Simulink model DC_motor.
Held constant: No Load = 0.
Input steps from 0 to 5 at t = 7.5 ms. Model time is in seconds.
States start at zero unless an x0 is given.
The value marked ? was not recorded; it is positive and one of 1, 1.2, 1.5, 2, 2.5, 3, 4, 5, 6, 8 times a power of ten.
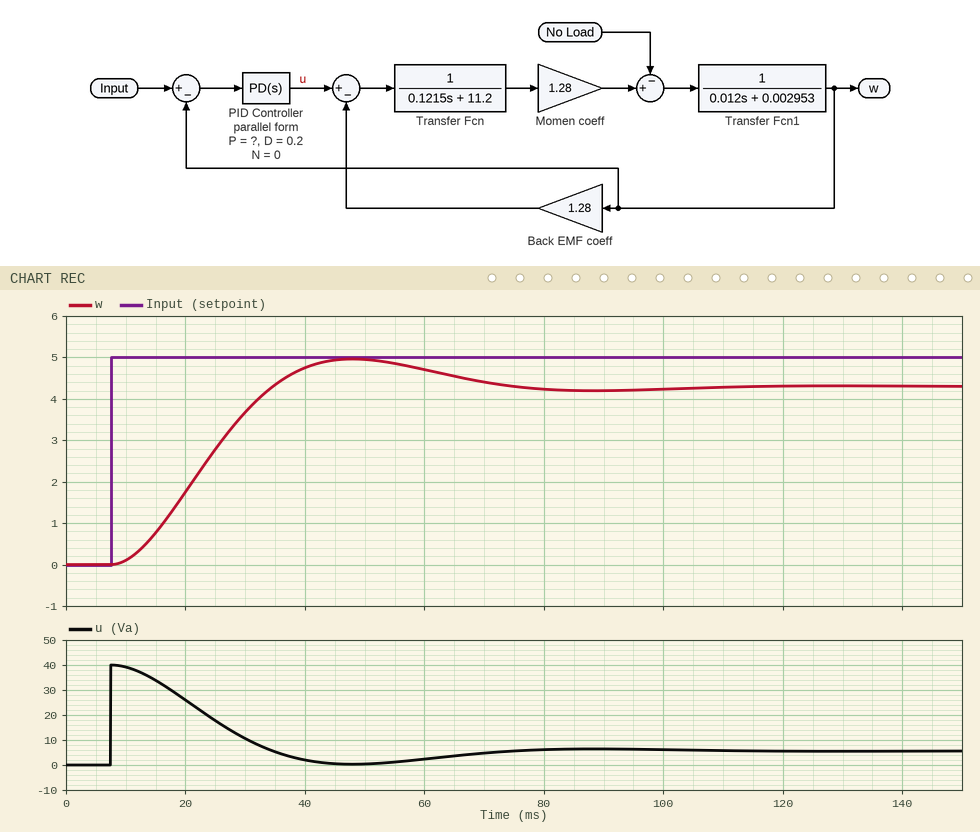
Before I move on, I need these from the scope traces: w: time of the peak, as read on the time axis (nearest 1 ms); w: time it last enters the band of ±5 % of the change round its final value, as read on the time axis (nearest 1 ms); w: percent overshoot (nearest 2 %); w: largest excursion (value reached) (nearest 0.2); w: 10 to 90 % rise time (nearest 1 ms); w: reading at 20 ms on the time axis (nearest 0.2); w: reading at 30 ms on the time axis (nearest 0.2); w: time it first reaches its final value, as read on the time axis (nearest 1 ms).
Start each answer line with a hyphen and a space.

- 48 ms
- 66 ms
- 16 %
- 5.0
- 18 ms
- 1.8
- 3.6
- 35 ms
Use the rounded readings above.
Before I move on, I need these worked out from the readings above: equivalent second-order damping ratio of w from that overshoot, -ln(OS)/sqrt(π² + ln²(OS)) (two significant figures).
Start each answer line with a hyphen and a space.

- 0.50
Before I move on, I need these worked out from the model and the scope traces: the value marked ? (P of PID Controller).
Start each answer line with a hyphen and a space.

- 8
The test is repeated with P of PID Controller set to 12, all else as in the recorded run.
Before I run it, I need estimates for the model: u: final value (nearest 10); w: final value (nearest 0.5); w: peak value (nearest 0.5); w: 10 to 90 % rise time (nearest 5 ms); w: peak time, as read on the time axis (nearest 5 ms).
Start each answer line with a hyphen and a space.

- 10
- 4.5
- 5.5
- 15 ms
- 40 ms
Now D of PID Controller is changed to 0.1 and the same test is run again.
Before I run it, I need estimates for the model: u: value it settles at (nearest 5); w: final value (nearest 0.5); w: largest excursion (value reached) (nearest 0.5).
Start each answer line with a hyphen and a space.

- 5
- 4.5
- 5.0
